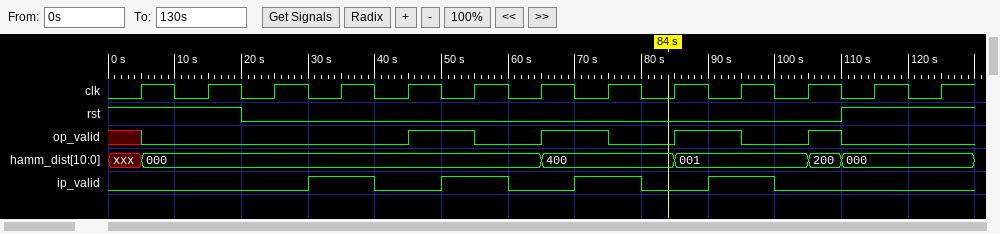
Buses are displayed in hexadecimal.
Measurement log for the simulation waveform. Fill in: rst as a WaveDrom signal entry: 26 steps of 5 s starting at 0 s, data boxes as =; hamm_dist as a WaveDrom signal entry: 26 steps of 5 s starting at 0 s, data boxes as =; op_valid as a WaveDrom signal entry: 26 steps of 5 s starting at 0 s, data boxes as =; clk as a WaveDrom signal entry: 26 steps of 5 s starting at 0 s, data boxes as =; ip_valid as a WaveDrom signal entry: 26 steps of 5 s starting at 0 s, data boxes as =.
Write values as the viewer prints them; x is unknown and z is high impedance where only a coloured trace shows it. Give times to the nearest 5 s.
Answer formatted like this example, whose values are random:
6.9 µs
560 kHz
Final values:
{name: 'rst', wave: '1...0.................1...'}
{name: 'hamm_dist', wave: 'x=...........=...=...==...', data: '000 400 001 200 000'}
{name: 'op_valid', wave: 'x0.......1.0.1.0.1.0.10...'}
{name: 'clk', wave: '01010101010101010101010101'}
{name: 'ip_valid', wave: '0.....1.0.1.0.1.0.1.0.....'}
